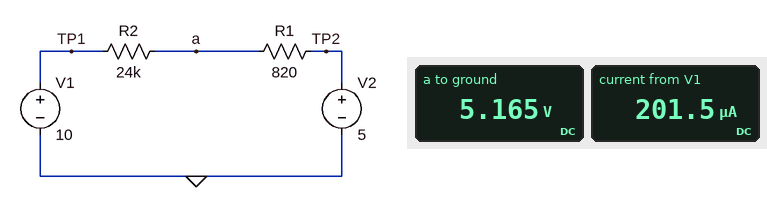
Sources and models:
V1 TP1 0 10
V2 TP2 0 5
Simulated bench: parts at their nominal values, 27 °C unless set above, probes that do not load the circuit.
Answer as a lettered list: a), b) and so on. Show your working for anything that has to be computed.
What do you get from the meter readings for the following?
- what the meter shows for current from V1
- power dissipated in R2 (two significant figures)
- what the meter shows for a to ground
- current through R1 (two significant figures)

a) 201.5 µA
b) (10 V - 5.165 V)^2 / 24 kΩ = 970 µW
c) 5.165 V
d) (5.165 V - 5 V) / 820 Ω = 200 µA
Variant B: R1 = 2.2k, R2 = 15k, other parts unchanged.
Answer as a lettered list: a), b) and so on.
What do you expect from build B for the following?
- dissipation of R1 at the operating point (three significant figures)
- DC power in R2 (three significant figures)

a) 186 µW
b) 1.27 mW
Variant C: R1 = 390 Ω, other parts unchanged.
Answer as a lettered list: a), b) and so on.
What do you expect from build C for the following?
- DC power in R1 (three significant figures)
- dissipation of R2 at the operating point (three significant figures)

a) 16.4 µW
b) 1.01 mW
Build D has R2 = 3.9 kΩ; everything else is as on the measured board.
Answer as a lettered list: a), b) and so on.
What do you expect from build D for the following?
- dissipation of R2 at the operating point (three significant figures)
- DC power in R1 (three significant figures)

a) 4.38 mW
b) 920 µW
